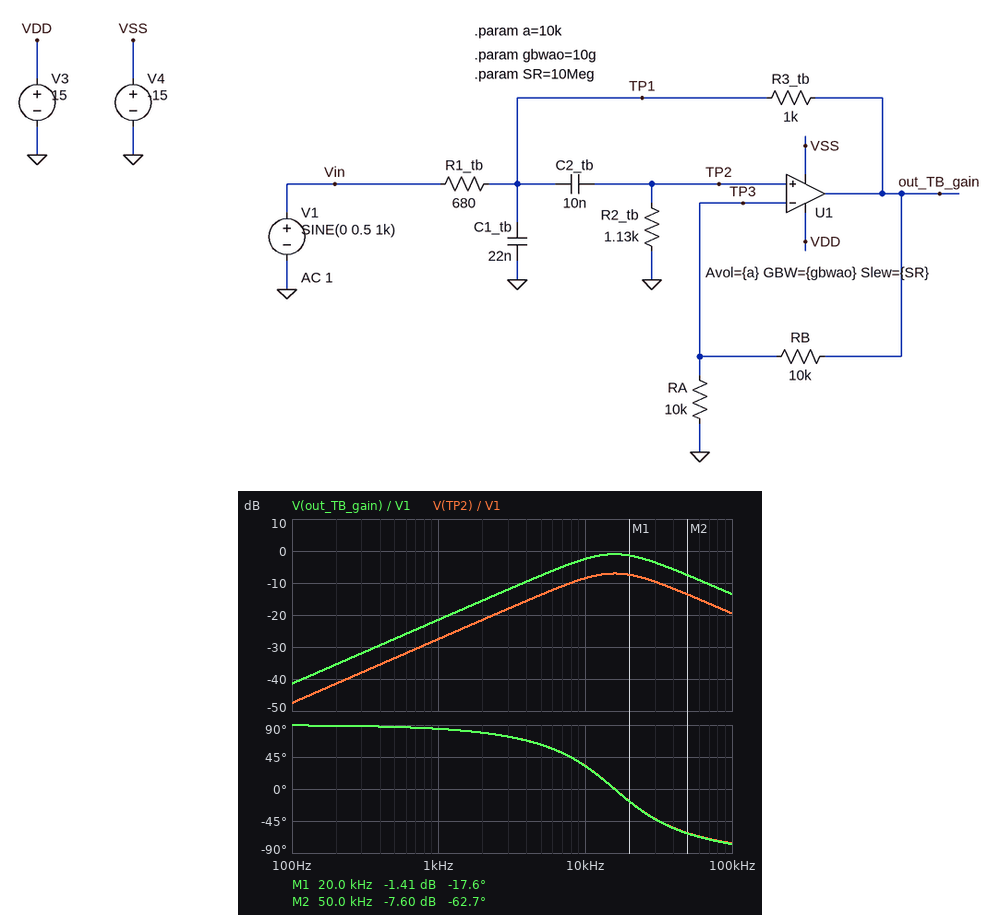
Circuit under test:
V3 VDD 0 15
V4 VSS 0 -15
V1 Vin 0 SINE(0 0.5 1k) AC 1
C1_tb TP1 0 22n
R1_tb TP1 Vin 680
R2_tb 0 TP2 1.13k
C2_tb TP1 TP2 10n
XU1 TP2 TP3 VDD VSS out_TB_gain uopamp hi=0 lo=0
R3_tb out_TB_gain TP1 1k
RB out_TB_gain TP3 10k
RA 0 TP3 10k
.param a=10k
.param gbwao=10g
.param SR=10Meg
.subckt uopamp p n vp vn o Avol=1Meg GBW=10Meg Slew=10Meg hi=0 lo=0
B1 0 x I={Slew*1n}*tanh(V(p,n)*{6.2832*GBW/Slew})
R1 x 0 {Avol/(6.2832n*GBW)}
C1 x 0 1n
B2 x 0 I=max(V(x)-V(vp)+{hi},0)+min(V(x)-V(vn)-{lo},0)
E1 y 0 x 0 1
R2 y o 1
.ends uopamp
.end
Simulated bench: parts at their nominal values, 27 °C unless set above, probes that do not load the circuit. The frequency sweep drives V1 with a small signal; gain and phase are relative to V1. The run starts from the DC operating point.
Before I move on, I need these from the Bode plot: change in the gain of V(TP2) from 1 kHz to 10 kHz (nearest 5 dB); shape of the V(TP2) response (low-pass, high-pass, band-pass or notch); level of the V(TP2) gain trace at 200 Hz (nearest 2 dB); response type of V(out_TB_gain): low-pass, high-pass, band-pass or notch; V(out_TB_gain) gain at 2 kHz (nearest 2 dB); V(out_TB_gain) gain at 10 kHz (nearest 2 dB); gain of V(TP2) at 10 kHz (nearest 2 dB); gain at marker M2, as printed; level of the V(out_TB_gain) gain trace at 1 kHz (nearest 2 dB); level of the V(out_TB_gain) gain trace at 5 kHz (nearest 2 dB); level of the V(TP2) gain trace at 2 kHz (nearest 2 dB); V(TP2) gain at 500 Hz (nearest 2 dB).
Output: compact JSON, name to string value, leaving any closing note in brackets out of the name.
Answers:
{"change in the gain of V(TP2) from 1 kHz to 10 kHz": "20 dB", "shape of the V(TP2) response": "band-pass", "level of the V(TP2) gain trace at 200 Hz": "-42 dB", "response type of V(out_TB_gain): low-pass, high-pass, band-pass or notch": "band-pass", "V(out_TB_gain) gain at 2 kHz": "-16 dB", "V(out_TB_gain) gain at 10 kHz": "-2 dB", "gain of V(TP2) at 10 kHz": "-8 dB", "gain at marker M2, as printed": "-7.60 dB", "level of the V(out_TB_gain) gain trace at 1 kHz": "-22 dB", "level of the V(out_TB_gain) gain trace at 5 kHz": "-8 dB", "level of the V(TP2) gain trace at 2 kHz": "-22 dB", "V(TP2) gain at 500 Hz": "-34 dB"}
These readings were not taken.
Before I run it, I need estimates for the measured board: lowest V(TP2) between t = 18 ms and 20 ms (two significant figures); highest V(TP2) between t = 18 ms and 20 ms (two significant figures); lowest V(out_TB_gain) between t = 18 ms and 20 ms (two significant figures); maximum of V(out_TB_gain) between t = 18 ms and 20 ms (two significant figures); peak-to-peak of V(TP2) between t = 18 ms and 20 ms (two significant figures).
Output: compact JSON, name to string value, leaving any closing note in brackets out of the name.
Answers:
{"lowest V(TP2) between t = 18 ms and 20 ms": "-21 mV", "highest V(TP2) between t = 18 ms and 20 ms": "21 mV", "lowest V(out_TB_gain) between t = 18 ms and 20 ms": "-42 mV", "maximum of V(out_TB_gain) between t = 18 ms and 20 ms": "42 mV", "peak-to-peak of V(TP2) between t = 18 ms and 20 ms": "42 mV"}
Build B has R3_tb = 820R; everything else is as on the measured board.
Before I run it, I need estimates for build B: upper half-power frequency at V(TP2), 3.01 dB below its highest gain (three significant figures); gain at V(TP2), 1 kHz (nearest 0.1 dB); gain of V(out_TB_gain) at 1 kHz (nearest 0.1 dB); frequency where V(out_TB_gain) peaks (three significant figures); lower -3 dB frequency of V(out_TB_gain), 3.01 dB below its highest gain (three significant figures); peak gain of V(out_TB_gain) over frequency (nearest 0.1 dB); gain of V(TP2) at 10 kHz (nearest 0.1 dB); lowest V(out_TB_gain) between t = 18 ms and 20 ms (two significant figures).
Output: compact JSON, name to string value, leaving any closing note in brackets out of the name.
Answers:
{"upper half-power frequency at V(TP2), 3.01 dB below its highest gain": "31.0 kHz", "gain at V(TP2), 1 kHz": "-28.2 dB", "gain of V(out_TB_gain) at 1 kHz": "-22.2 dB", "frequency where V(out_TB_gain) peaks": "16.5 kHz", "lower -3 dB frequency of V(out_TB_gain), 3.01 dB below its highest gain": "8.80 kHz", "peak gain of V(out_TB_gain) over frequency": "-0.4 dB", "gain of V(TP2) at 10 kHz": "-8.5 dB", "lowest V(out_TB_gain) between t = 18 ms and 20 ms": "-39 mV"}
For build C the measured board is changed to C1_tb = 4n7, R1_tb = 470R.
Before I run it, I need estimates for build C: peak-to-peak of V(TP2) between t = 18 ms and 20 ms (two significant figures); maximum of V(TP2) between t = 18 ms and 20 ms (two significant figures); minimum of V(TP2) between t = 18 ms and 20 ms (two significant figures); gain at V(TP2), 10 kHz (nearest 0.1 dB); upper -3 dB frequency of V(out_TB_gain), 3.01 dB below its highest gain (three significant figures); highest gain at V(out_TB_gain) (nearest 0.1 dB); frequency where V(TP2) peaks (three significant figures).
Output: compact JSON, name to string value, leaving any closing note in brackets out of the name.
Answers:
{"peak-to-peak of V(TP2) between t = 18 ms and 20 ms": "48 mV", "maximum of V(TP2) between t = 18 ms and 20 ms": "24 mV", "minimum of V(TP2) between t = 18 ms and 20 ms": "-24 mV", "gain at V(TP2), 10 kHz": "-7.0 dB", "upper -3 dB frequency of V(out_TB_gain), 3.01 dB below its highest gain": "96.4 kHz", "highest gain at V(out_TB_gain)": "4.9 dB", "frequency where V(TP2) peaks": "38.4 kHz"}
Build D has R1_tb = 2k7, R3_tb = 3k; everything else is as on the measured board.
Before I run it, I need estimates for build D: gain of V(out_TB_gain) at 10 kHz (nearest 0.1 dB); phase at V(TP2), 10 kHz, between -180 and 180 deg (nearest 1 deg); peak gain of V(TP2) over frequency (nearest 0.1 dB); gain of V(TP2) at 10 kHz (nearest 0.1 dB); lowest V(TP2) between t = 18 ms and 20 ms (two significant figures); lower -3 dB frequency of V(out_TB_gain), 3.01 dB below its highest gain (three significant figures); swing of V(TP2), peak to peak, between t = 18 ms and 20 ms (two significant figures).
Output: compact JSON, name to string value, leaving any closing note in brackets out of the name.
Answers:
{"gain of V(out_TB_gain) at 10 kHz": "-11.8 dB", "phase at V(TP2), 10 kHz, between -180 and 180 deg": "-8 deg", "peak gain of V(TP2) over frequency": "-17.8 dB", "gain of V(TP2) at 10 kHz": "-17.9 dB", "lowest V(TP2) between t = 18 ms and 20 ms": "-18 mV", "lower -3 dB frequency of V(out_TB_gain), 3.01 dB below its highest gain": "3.02 kHz", "swing of V(TP2), peak to peak, between t = 18 ms and 20 ms": "36 mV"}
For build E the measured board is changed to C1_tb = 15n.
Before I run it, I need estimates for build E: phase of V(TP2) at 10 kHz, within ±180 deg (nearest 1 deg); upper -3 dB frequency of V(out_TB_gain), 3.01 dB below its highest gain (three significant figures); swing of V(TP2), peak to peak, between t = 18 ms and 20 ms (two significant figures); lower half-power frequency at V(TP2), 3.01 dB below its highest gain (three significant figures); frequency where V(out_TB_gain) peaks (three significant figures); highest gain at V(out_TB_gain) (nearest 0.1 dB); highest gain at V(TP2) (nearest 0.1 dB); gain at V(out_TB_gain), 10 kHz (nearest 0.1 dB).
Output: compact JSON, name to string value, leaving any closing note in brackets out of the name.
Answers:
{"phase of V(TP2) at 10 kHz, within ±180 deg": "43 deg", "upper -3 dB frequency of V(out_TB_gain), 3.01 dB below its highest gain": "38.0 kHz", "swing of V(TP2), peak to peak, between t = 18 ms and 20 ms": "42 mV", "lower half-power frequency at V(TP2), 3.01 dB below its highest gain": "9.67 kHz", "frequency where V(out_TB_gain) peaks": "19.2 kHz", "highest gain at V(out_TB_gain)": "0.8 dB", "highest gain at V(TP2)": "-5.2 dB", "gain at V(out_TB_gain), 10 kHz": "-2.0 dB"}
